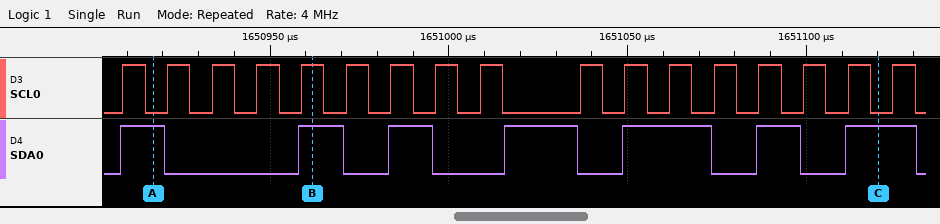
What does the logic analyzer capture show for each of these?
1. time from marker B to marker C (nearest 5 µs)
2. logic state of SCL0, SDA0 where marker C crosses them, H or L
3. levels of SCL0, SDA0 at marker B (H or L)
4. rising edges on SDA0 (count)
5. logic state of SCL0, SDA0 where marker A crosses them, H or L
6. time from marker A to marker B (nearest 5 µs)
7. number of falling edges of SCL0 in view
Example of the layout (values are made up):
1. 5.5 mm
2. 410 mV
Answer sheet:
1. 160 µs
2. SCL0=L, SDA0=H
3. SCL0=H, SDA0=H
4. 7
5. SCL0=L, SDA0=H
6. 45 µs
7. 17
